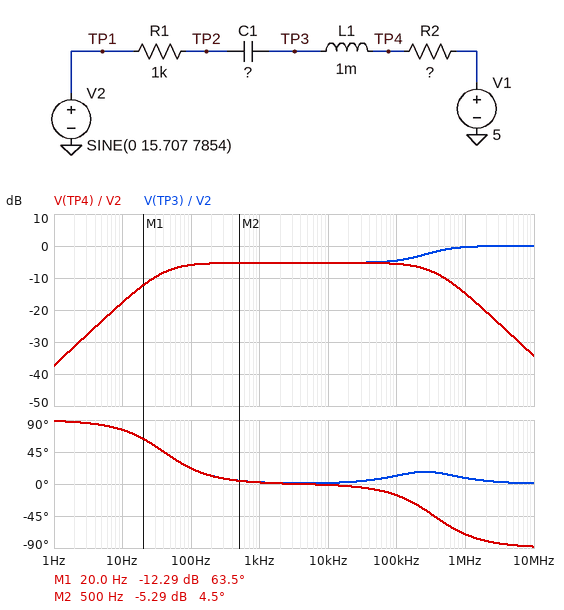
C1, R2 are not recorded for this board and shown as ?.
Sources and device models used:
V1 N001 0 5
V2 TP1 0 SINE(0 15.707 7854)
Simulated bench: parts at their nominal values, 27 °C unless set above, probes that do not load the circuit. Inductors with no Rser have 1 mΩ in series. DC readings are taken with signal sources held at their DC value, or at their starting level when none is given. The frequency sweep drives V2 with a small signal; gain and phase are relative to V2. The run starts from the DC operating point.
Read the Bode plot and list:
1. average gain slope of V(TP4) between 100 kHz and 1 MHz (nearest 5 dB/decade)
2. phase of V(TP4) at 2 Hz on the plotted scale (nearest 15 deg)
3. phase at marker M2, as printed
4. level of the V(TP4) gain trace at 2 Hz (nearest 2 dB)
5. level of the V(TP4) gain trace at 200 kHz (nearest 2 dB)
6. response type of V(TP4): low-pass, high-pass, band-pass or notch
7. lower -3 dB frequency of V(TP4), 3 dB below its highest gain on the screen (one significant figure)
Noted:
-10 dB/decade
90 deg
4.5 deg
-32 dB
-6 dB
band-pass
40 Hz
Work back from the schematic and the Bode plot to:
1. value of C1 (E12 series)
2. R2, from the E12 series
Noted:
1.8 µF
1.2 kΩ
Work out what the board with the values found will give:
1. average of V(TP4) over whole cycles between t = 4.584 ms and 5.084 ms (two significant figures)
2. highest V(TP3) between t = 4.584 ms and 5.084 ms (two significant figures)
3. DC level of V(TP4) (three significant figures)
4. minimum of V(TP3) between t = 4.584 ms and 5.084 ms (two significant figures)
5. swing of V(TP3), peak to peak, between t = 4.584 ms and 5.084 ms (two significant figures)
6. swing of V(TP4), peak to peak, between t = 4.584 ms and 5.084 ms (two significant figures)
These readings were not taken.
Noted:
5.0 V
14 V
5.00 V
-3.6 V
17 V
17 V
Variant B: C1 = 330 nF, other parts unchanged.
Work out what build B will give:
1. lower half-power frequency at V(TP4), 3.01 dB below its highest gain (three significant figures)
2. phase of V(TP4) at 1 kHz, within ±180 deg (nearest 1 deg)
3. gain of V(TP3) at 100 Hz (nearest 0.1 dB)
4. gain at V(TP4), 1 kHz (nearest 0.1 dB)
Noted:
219 Hz
12 deg
-12.9 dB
-5.5 dB
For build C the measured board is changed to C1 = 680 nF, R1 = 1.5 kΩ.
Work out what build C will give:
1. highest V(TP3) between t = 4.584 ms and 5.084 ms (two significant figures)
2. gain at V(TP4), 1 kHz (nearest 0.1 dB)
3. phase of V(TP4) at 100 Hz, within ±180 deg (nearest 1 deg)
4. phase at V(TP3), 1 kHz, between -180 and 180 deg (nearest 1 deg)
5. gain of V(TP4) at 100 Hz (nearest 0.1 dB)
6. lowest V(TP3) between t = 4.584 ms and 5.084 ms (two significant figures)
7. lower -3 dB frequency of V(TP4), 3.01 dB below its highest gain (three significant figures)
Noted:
12 V
-7.1 dB
41 deg
5 deg
-9.5 dB
-2.0 V
86.7 Hz
